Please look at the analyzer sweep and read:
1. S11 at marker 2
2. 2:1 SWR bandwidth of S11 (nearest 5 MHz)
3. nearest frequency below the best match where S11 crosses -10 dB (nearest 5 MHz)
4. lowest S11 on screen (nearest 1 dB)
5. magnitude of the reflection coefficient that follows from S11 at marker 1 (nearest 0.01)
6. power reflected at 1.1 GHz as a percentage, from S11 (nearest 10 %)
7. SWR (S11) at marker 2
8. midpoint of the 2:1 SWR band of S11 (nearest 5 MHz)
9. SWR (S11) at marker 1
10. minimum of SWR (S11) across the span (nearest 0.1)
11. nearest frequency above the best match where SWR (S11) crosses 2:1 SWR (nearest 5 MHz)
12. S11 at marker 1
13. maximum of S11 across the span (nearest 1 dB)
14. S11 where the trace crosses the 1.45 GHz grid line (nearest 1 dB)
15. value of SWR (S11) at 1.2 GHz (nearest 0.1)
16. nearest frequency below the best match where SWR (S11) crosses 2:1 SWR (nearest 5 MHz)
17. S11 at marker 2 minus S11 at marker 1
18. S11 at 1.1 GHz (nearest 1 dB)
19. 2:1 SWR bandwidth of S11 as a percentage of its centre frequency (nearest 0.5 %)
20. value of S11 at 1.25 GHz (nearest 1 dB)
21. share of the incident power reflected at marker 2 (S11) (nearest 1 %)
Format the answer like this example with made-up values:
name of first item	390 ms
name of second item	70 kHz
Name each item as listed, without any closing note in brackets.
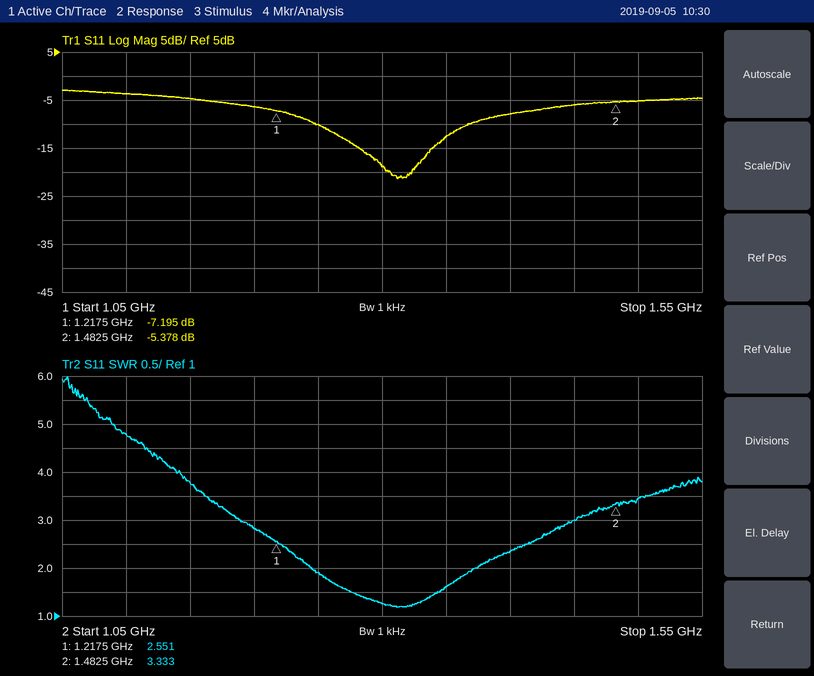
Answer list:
S11 at marker 2	-5.378 dB
2:1 SWR bandwidth of S11	130 MHz
nearest frequency below the best match where S11 crosses -10 dB	1.250 GHz
lowest S11 on screen	-21 dB
magnitude of the reflection coefficient that follows from S11 at marker 1	0.44
power reflected at 1.1 GHz as a percentage, from S11	40 %
SWR (S11) at marker 2	3.333
midpoint of the 2:1 SWR band of S11	1.310 GHz
SWR (S11) at marker 1	2.551
minimum of SWR (S11) across the span	1.2
nearest frequency above the best match where SWR (S11) crosses 2:1 SWR	1.375 GHz
S11 at marker 1	-7.195 dB
maximum of S11 across the span	-3 dB
S11 where the trace crosses the 1.45 GHz grid line	-6 dB
value of SWR (S11) at 1.2 GHz	2.8
nearest frequency below the best match where SWR (S11) crosses 2:1 SWR	1.245 GHz
S11 at marker 2 minus S11 at marker 1	1.817 dB
S11 at 1.1 GHz	-4 dB
2:1 SWR bandwidth of S11 as a percentage of its centre frequency	10.0 %
value of S11 at 1.25 GHz	-10 dB
share of the incident power reflected at marker 2 (S11)	29 %
